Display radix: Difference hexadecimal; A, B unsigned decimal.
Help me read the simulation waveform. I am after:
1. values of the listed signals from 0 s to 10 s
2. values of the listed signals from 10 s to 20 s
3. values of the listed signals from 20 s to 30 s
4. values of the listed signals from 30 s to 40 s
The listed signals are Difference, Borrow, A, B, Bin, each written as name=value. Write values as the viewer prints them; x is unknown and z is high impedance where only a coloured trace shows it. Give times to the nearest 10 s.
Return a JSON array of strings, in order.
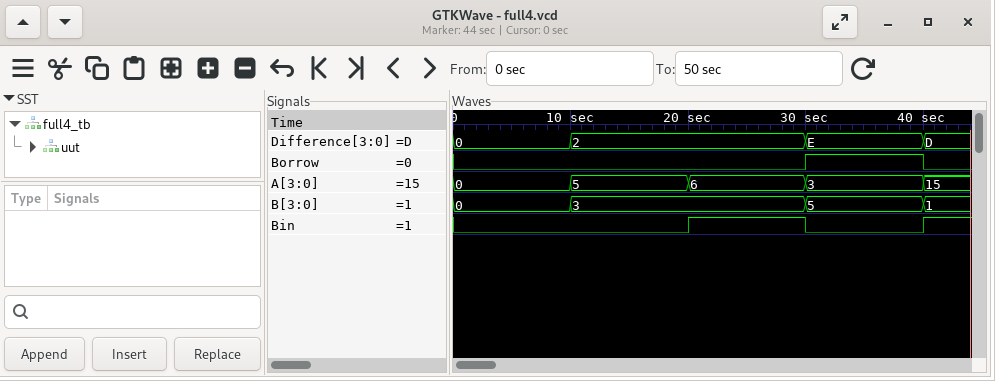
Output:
["Difference=0, Borrow=0, A=0, B=0, Bin=0", "Difference=2, Borrow=0, A=5, B=3, Bin=0", "Difference=2, Borrow=0, A=6, B=3, Bin=1", "Difference=E, Borrow=1, A=3, B=5, Bin=0"]
